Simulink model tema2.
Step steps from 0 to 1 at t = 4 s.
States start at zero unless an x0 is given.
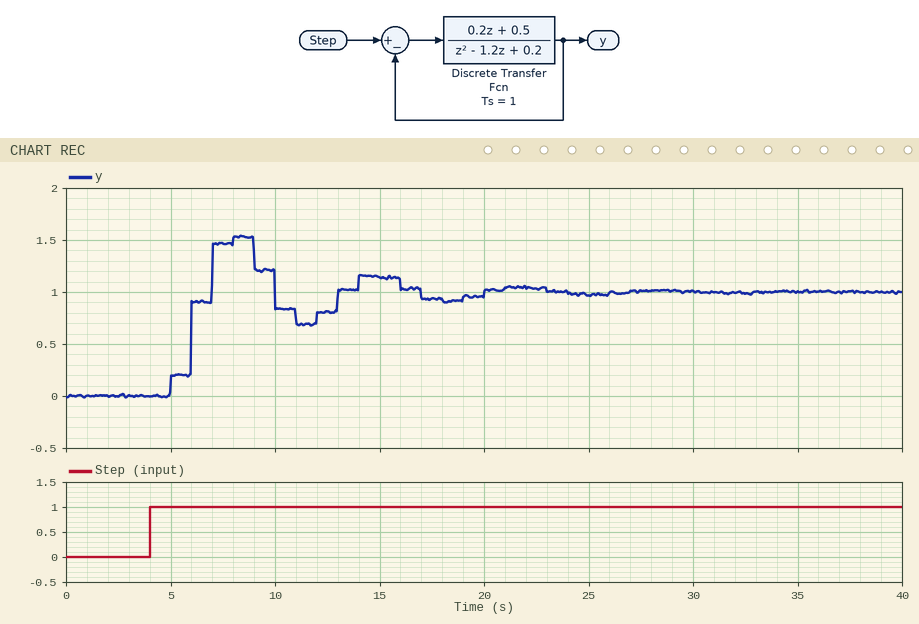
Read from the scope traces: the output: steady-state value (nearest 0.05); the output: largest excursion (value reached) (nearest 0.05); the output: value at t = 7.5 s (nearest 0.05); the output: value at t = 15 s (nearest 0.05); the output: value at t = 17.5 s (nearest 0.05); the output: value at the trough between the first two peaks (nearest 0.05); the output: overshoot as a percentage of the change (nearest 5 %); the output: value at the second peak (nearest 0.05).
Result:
1.00
1.55
1.45
1.15
0.95
0.70
55 %
1.15
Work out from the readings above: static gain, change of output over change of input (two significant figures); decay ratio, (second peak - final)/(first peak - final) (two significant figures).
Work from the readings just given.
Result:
1.0
0.27
